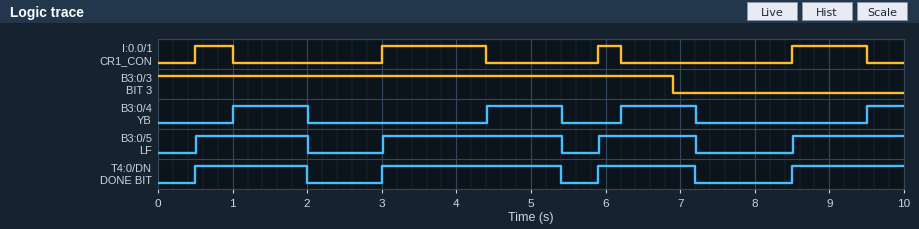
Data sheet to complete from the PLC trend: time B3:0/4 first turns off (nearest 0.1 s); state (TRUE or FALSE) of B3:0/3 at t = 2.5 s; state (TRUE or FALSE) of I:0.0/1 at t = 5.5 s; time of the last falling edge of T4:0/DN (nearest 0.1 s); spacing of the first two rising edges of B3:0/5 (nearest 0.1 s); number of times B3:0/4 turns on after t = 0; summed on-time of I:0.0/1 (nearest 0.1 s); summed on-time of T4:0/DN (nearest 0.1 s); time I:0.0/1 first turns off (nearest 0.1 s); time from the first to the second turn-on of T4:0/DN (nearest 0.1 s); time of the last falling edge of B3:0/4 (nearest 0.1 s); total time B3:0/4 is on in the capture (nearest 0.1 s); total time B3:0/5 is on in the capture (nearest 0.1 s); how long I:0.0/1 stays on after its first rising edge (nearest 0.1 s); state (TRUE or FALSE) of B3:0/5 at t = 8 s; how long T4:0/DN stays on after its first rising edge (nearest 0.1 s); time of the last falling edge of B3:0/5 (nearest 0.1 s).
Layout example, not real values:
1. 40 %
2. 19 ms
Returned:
1. 2.0 s
2. TRUE
3. FALSE
4. 7.2 s
5. 2.5 s
6. 4
7. 3.2 s
8. 6.7 s
9. 1.0 s
10. 2.5 s
11. 7.2 s
12. 3.5 s
13. 6.7 s
14. 0.5 s
15. FALSE
16. 1.5 s
17. 7.2 s
